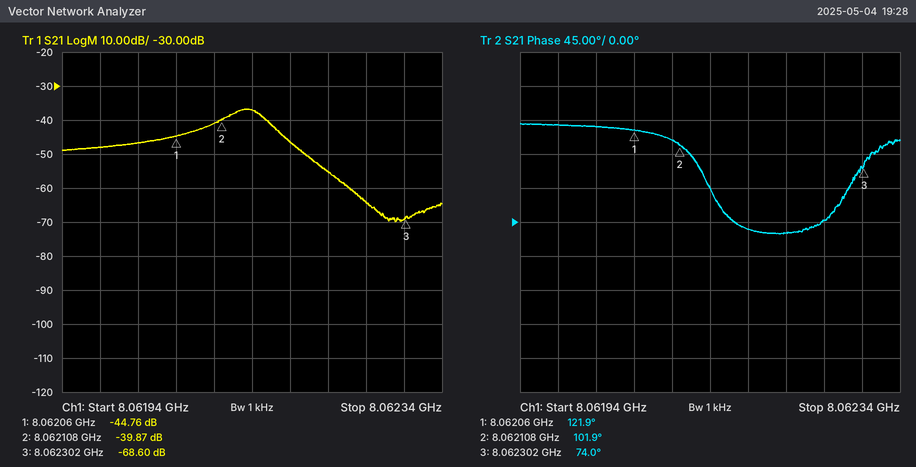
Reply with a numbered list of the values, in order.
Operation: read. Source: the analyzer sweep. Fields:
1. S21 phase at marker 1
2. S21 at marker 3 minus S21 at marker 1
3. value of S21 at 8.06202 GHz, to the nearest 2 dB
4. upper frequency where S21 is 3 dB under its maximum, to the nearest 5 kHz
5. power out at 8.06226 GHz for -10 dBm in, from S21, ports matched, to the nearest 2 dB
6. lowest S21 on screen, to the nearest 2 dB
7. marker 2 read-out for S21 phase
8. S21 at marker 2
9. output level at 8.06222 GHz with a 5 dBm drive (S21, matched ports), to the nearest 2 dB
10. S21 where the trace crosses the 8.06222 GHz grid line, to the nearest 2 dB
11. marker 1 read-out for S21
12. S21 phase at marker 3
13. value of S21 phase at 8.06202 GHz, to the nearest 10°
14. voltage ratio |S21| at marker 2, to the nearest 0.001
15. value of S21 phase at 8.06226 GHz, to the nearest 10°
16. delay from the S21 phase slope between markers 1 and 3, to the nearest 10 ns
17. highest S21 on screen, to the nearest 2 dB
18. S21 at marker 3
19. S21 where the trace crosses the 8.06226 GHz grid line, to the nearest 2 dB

1. 121.9°
2. -23.84 dB
3. -46 dB
4. 8.062155 GHz
5. -74 dBm
6. -70 dB
7. 101.9°
8. -39.87 dB
9. -50 dBm
10. -56 dB
11. -44.76 dB
12. 74.0°
13. 130°
14. 0.010
15. 0°
16. 550 ns
17. -36 dB
18. -68.60 dB
19. -64 dB
